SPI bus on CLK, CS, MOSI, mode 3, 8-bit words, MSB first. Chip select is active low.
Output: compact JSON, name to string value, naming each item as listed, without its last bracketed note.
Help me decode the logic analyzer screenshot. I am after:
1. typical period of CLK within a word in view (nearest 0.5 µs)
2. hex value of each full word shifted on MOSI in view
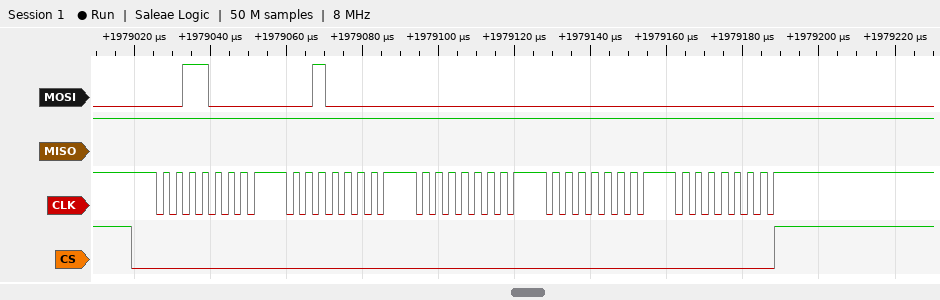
{"typical period of CLK within a word in view": "3.5 µs", "hex value of each full word shifted on MOSI in view": "30, 20, 00, 00, 00"}
